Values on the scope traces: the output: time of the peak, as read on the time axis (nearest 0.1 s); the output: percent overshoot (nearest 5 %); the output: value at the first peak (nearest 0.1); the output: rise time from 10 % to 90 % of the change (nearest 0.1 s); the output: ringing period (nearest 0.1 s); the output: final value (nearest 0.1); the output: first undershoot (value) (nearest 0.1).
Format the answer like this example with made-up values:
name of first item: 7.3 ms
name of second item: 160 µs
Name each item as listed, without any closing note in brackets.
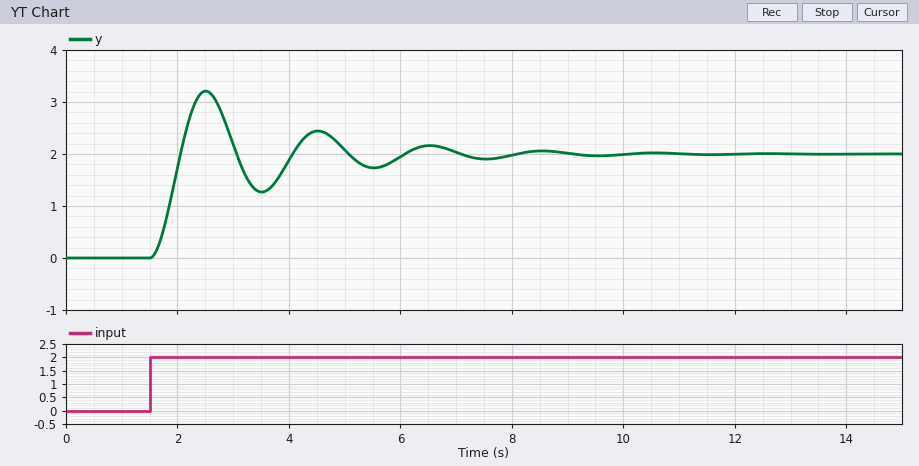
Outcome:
the output: time of the peak, as read on the time axis: 2.5 s
the output: percent overshoot: 60 %
the output: value at the first peak: 3.2
the output: rise time from 10 % to 90 % of the change: 0.4 s
the output: ringing period: 2.0 s
the output: final value: 2.0
the output: first undershoot (value): 1.3
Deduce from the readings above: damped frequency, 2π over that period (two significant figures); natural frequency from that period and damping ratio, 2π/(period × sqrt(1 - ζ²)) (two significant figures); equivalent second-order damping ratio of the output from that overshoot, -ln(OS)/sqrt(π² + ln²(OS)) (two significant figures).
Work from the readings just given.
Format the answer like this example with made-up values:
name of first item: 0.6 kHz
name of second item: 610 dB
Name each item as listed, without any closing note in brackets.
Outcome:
damped frequency, 2π over that period: 3.1 rad/s
natural frequency from that period and damping ratio, 2π/(period × sqrt(1 - ζ²)): 3.2 rad/s
equivalent second-order damping ratio of the output from that overshoot, -ln(OS)/sqrt(π² + ln²(OS)): 0.16
